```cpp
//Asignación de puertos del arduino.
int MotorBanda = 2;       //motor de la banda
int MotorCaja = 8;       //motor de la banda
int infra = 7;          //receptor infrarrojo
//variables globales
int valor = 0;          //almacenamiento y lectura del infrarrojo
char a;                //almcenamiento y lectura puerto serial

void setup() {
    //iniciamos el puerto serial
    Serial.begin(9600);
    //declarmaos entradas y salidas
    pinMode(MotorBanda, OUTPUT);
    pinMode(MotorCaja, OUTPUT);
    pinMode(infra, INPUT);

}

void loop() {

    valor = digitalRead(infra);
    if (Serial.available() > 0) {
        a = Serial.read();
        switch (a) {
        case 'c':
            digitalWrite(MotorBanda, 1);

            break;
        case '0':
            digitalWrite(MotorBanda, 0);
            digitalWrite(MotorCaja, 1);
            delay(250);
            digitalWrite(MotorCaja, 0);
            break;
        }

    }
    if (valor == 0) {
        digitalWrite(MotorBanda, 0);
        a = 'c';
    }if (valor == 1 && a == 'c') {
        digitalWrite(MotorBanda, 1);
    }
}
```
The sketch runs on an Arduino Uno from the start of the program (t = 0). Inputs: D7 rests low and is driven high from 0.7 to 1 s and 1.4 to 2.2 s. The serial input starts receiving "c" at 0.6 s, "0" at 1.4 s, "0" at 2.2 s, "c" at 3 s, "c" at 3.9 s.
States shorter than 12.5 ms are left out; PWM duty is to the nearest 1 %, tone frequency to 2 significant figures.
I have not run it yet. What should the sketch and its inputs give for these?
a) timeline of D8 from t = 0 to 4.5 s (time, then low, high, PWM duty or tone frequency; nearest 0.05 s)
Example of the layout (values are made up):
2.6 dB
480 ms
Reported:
0 s low; 1.4 s high; 1.65 s low; 2.2 s high; 2.45 s low
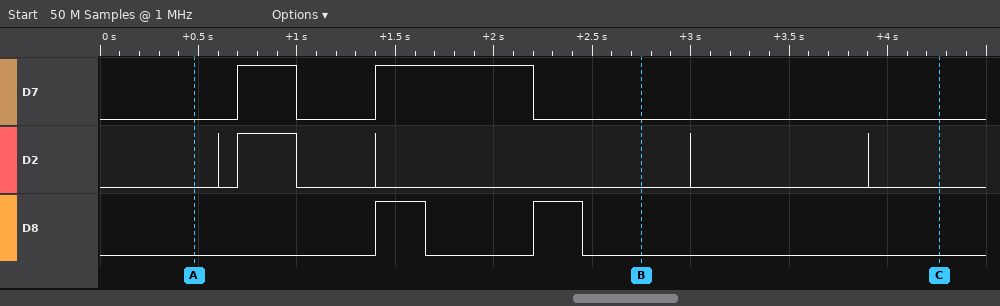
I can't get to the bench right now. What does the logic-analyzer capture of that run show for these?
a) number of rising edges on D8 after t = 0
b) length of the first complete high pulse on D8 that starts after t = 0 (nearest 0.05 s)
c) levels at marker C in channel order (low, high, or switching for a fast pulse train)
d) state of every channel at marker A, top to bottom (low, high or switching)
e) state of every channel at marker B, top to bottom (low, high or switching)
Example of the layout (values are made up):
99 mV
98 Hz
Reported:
2
0.25 s
D7 low, D2 low, D8 low
D7 low, D2 low, D8 low
D7 low, D2 low, D8 low
